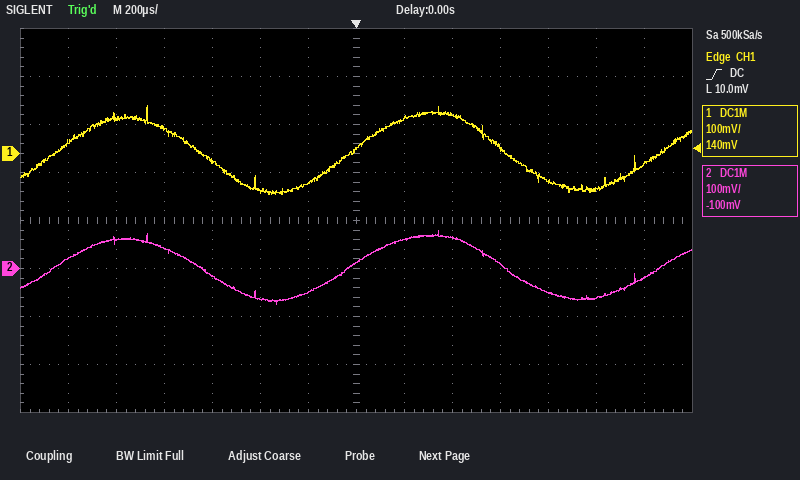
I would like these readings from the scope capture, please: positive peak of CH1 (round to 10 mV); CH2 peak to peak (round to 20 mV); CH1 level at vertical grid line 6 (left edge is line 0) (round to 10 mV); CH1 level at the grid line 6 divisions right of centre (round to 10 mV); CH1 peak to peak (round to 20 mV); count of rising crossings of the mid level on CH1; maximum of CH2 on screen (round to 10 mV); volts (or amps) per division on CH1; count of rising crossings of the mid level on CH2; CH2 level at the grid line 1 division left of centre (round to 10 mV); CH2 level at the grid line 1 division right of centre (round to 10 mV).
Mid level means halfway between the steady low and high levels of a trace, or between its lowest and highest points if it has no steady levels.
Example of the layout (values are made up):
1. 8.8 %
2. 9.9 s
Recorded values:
1. 100 mV
2. 160 mV
3. -60 mV
4. -20 mV
5. 180 mV
6. 3
7. 80 mV
8. 100 mV
9. 3
10. -50 mV
11. 60 mV
